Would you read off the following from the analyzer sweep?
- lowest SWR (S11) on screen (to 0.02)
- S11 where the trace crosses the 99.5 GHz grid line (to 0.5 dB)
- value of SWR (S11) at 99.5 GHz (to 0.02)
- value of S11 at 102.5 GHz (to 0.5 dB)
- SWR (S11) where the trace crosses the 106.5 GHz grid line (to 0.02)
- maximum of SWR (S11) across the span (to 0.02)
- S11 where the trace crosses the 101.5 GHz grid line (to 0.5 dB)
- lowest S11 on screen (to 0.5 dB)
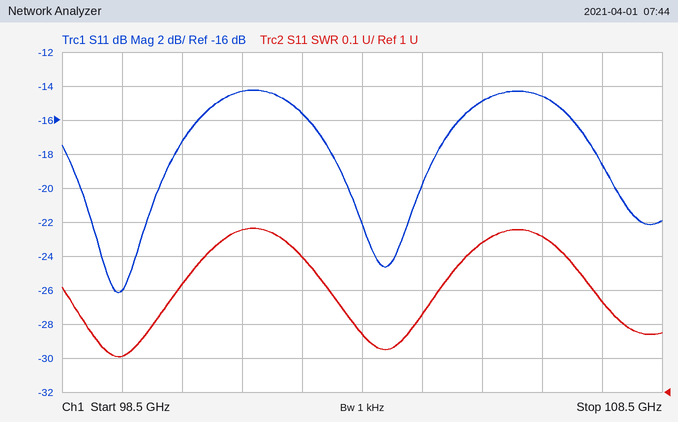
1.10
-26.0 dB
1.10
-15.5 dB
1.46
1.48
-14.5 dB
-26.0 dB
